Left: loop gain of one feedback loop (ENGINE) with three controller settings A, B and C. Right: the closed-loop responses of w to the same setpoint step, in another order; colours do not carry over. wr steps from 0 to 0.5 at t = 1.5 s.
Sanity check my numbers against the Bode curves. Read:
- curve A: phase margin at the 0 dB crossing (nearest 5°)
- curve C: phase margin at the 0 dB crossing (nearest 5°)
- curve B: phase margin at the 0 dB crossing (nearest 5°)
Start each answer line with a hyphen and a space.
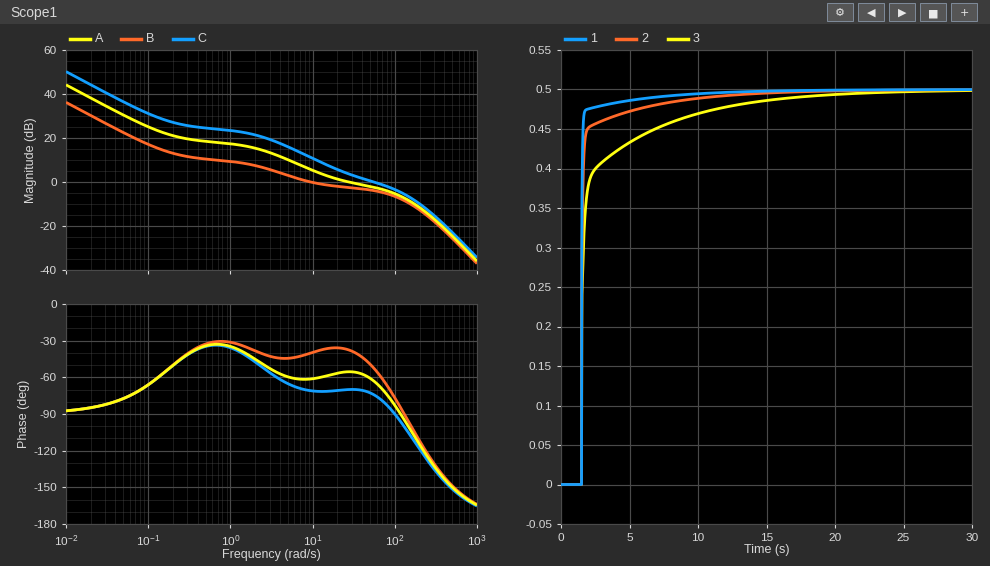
- 125°
- 105°
- 140°
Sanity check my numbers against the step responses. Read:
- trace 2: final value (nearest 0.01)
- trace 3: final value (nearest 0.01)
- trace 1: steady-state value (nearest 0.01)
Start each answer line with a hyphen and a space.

- 0.50
- 0.50
- 0.50
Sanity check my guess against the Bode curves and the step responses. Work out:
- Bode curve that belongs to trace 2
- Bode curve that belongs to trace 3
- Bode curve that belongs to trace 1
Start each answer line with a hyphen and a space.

- A
- B
- C
